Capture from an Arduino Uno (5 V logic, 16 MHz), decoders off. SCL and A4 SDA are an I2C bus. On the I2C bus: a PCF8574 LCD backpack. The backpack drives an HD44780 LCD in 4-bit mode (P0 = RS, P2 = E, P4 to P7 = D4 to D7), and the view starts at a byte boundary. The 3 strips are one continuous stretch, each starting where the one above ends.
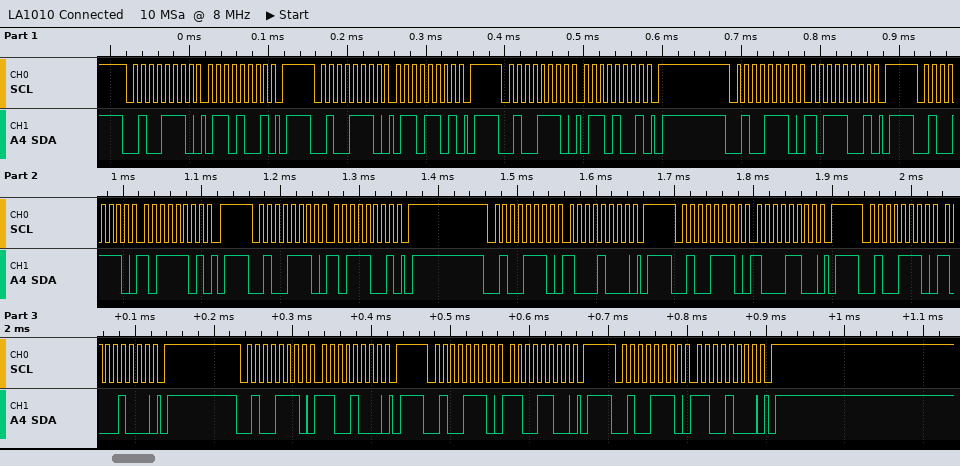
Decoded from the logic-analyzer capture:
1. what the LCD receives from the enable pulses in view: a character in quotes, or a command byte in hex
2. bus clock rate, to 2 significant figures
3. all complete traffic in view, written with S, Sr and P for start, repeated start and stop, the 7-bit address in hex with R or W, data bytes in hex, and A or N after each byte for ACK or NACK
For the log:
'k' 0x8C
100 kHz
S 27W A 69 A P S 27W A 6D A P S 27W A 69 A P S 27W A B9 A P S 27W A BD A P S 27W A B9 A P S 27W A 88 A P S 27W A 8C A P S 27W A 88 A P S 27W A C8 A P S 27W A CC A P S 27W A C8 A P
